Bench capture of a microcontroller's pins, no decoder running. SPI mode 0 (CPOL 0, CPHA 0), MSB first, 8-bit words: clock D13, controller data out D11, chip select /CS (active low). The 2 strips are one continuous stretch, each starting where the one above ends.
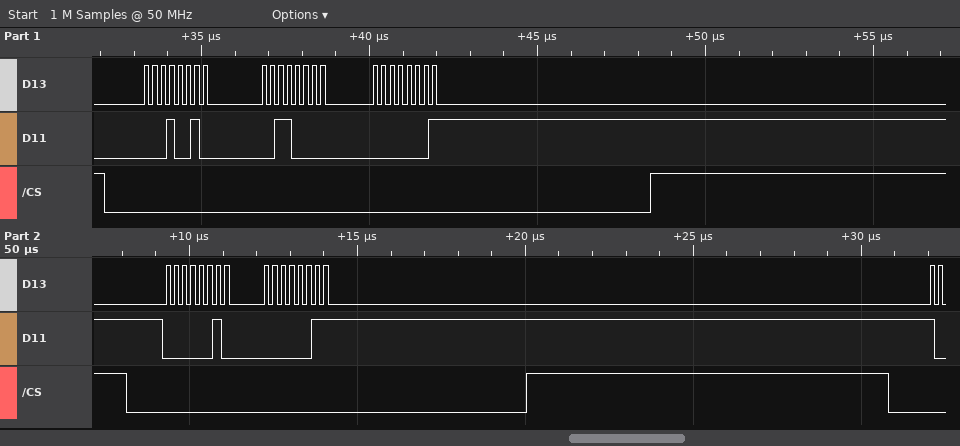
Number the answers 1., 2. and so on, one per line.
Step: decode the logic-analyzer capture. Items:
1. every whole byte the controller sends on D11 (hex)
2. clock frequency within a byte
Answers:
1. 12 30 01 02 03
2. 4 MHz
